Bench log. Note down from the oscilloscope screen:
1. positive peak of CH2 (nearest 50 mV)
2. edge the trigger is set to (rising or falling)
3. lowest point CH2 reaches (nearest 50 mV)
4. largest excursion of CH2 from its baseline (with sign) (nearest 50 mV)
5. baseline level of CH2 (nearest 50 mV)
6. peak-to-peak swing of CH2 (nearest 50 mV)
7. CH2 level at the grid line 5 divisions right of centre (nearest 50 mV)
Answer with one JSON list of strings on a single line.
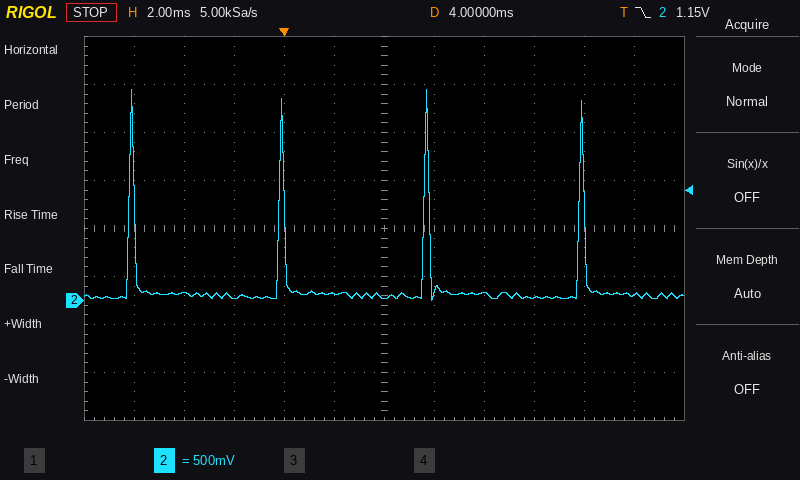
["2.20 V", "falling", "0 mV", "+2.15 V", "50 mV", "2.20 V", "50 mV"]
